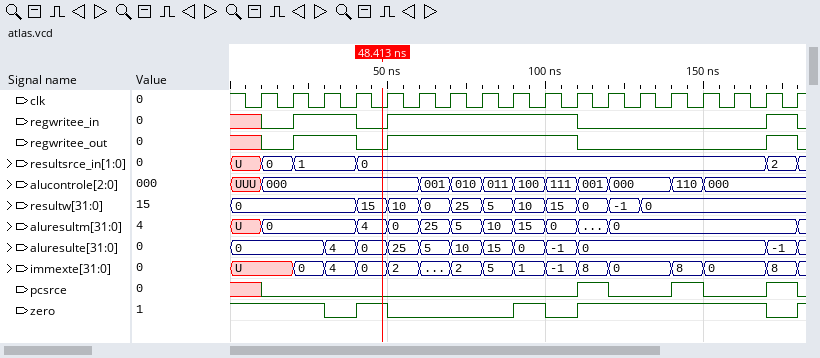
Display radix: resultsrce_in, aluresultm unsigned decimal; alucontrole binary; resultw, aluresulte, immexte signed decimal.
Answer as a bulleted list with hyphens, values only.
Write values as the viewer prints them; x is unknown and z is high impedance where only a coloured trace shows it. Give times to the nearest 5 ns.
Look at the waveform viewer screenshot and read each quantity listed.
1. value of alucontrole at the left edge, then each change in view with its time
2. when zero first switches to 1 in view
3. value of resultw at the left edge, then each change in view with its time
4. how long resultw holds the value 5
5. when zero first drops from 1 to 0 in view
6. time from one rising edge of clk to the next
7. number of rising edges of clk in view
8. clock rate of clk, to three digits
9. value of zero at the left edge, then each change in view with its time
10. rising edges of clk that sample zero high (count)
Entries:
- UUU, 000 at 10 ns, 001 at 60 ns, 010 at 70 ns, 011 at 80 ns, 100 at 90 ns, 111 at 100 ns, 001 at 110 ns, 000 at 120 ns, 110 at 140 ns, 000 at 150 ns
- 40 ns
- 0, 15 at 40 ns, 10 at 50 ns, 0 at 60 ns, 25 at 70 ns, 5 at 80 ns, 10 at 90 ns, 15 at 100 ns, 0 at 110 ns, -1 at 120 ns, 0 at 130 ns
- 10 ns
- 30 ns
- 10 ns
- 18
- 100 MHz
- 1, 0 at 30 ns, 1 at 40 ns, 0 at 50 ns, 1 at 90 ns, 0 at 100 ns, 1 at 110 ns, 0 at 170 ns, 1 at 180 ns
- 11
